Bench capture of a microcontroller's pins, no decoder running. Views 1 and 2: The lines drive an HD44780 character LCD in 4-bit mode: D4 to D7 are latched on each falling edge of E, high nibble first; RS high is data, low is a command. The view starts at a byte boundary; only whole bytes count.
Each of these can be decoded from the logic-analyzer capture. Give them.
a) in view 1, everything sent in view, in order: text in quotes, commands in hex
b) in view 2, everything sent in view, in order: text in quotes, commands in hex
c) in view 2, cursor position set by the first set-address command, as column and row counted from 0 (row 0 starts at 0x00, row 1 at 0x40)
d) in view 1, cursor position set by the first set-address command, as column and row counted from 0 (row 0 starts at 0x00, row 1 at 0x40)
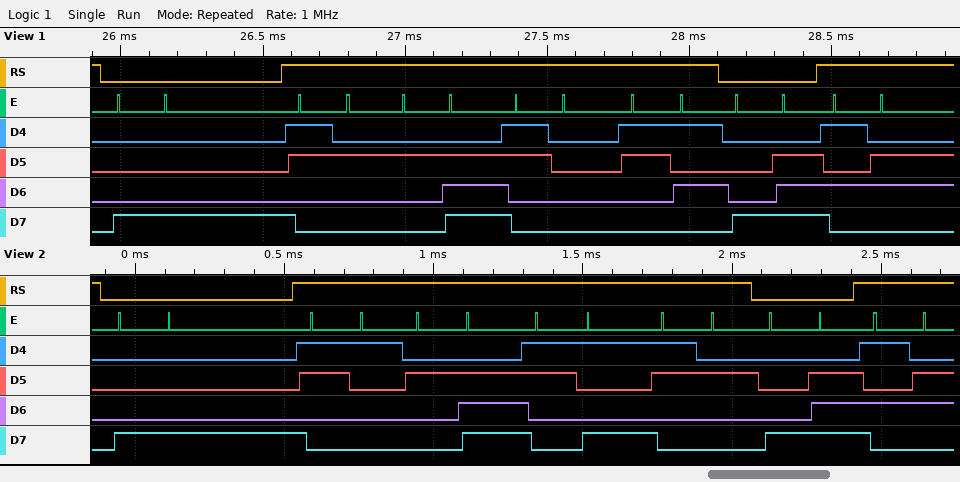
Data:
0x88 "2.05" 0x8E "V"
0x88 "1.92" 0x8E "V"
column 8, row 0
column 8, row 0
